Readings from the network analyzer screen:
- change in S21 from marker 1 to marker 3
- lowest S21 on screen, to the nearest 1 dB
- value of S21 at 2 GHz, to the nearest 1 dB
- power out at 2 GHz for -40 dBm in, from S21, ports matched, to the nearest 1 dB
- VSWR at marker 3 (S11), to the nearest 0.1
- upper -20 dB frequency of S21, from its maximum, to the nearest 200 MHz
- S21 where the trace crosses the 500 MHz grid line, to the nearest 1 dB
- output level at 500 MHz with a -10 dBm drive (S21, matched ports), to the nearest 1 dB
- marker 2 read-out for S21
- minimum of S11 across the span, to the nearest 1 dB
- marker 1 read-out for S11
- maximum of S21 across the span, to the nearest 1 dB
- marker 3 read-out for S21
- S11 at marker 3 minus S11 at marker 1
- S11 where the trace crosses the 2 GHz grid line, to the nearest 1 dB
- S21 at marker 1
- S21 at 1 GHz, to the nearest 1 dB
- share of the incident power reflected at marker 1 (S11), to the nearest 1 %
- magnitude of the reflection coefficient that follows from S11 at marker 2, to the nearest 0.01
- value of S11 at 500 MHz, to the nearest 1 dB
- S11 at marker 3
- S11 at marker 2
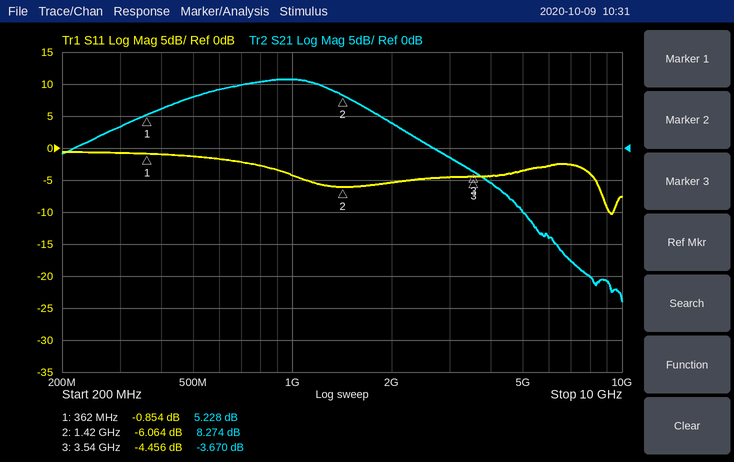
-8.898 dB
-24 dB
4 dB
-36 dBm
4.0
4.8 GHz
8 dB
-2 dBm
8.274 dB
-10 dB
-0.854 dB
11 dB
-3.670 dB
-3.602 dB
-5 dB
5.228 dB
11 dB
82 %
0.50
-1 dB
-4.456 dB
-6.064 dB
